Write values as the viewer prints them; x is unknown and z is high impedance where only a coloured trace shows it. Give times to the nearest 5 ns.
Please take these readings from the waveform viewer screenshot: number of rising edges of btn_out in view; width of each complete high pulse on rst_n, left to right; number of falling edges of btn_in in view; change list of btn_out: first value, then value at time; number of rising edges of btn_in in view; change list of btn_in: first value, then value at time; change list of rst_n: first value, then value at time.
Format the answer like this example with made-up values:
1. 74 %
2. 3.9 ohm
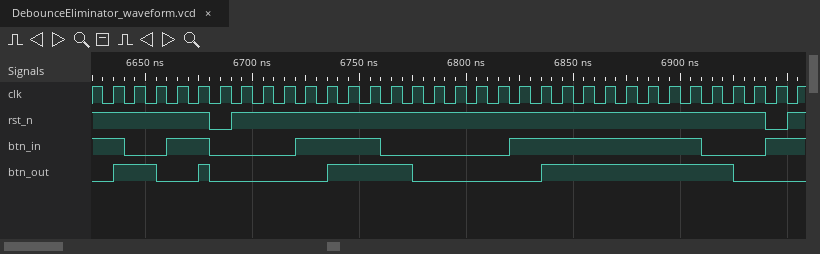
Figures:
1. 4
2. 250 ns
3. 4
4. 0, 1 at 6635 ns, 0 at 6655 ns, 1 at 6675 ns, 0 at 6680 ns, 1 at 6735 ns, 0 at 6775 ns, 1 at 6835 ns, 0 at 6925 ns
5. 4
6. 1, 0 at 6640 ns, 1 at 6660 ns, 0 at 6680 ns, 1 at 6720 ns, 0 at 6760 ns, 1 at 6820 ns, 0 at 6910 ns, 1 at 6940 ns
7. 1, 0 at 6680 ns, 1 at 6690 ns, 0 at 6940 ns, 1 at 6950 ns
